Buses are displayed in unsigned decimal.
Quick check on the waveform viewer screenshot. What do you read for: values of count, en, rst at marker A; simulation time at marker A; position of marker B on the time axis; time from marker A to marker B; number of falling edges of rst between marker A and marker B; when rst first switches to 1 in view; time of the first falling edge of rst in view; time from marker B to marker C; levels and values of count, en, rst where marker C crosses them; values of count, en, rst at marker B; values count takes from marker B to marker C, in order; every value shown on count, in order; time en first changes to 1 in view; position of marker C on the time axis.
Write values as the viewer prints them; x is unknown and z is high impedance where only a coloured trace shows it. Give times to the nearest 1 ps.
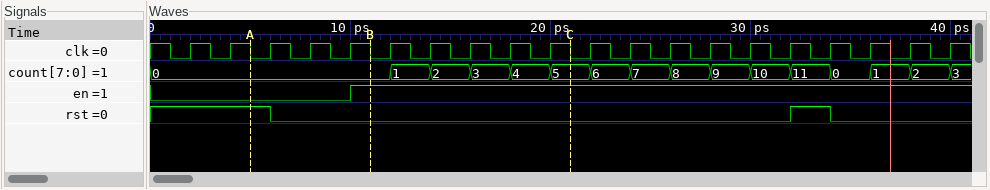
count=0, en=0, rst=1
5 ps
11 ps
6 ps
1
32 ps
6 ps
10 ps
count=5, en=1, rst=0
count=0, en=1, rst=0
0, 1, 2, 3, 4, 5
0, 1, 2, 3, 4, 5, 6, 7, 8, 9, 10, 11, 0, 1, 2, 3
10 ps
21 ps
